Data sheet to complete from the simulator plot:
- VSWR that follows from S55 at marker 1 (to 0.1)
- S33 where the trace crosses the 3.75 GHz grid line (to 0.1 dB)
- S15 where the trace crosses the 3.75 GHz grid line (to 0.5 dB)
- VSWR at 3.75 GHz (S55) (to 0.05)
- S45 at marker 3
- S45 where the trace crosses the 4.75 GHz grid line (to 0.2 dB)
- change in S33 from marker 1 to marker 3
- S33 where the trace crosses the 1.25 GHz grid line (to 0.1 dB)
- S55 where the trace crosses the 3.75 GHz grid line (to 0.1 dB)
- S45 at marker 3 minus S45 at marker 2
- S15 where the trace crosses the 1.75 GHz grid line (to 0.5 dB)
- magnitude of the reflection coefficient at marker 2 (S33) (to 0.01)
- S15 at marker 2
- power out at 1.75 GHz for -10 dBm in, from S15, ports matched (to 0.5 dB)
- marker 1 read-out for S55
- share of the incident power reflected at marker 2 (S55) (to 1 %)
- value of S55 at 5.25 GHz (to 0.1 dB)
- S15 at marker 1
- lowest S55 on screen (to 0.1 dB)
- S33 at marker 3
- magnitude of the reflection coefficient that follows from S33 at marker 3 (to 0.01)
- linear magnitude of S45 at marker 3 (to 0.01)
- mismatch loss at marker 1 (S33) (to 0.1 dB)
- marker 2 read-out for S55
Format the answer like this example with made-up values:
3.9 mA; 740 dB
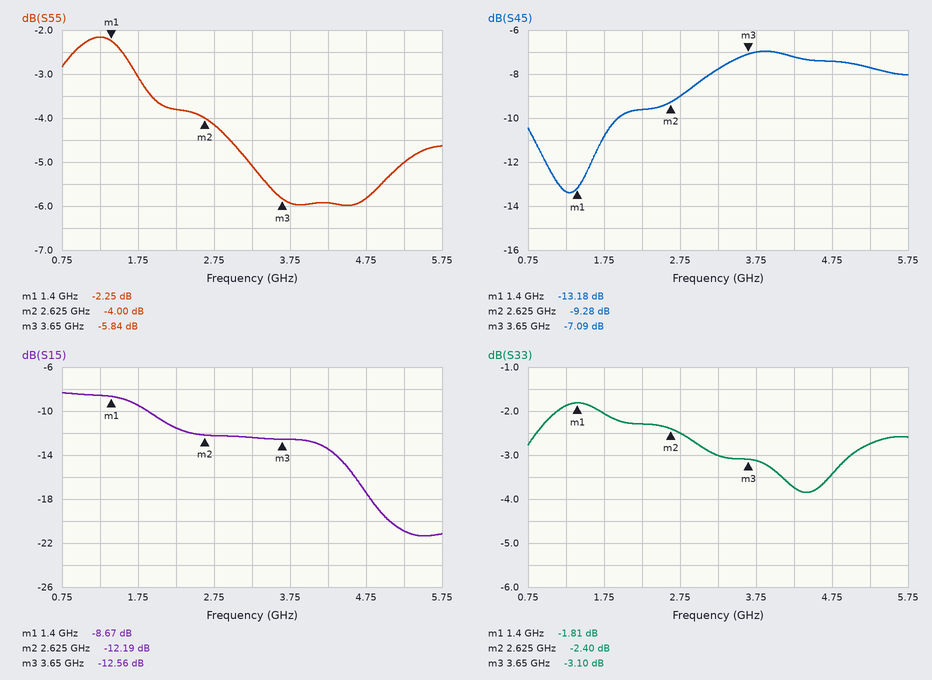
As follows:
7.8; -3.1 dB; -12.5 dB; 3.05; -7.09 dB; -7.4 dB; -1.29 dB; -1.9 dB; -5.9 dB; 2.19 dB; -9.5 dB; 0.76; -12.19 dB; -19.5 dBm; -2.25 dB; 40 %; -5.0 dB; -8.67 dB; -6.0 dB; -3.10 dB; 0.70; 0.44; 4.7 dB; -4.00 dB
